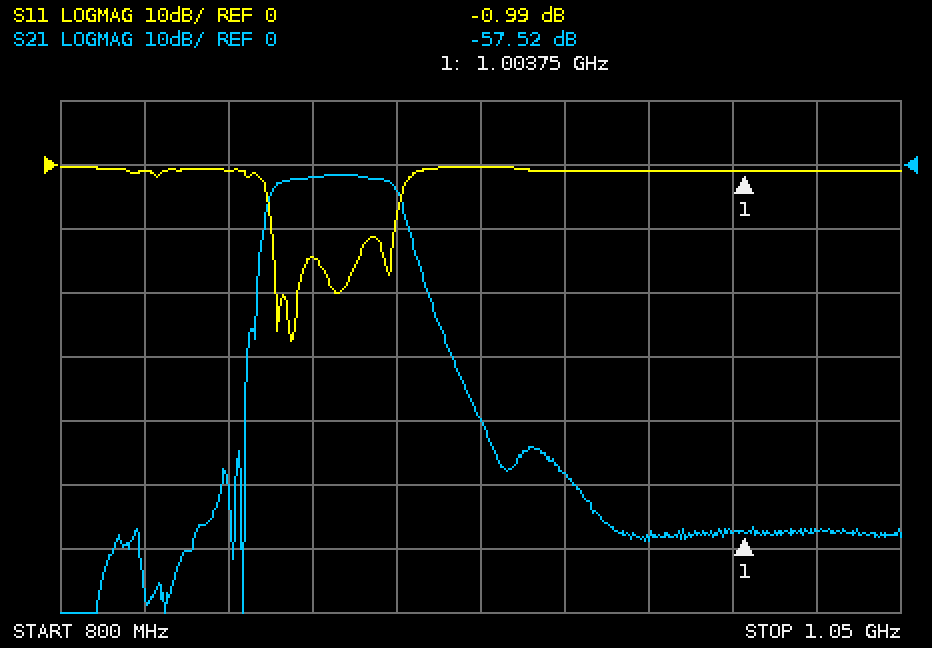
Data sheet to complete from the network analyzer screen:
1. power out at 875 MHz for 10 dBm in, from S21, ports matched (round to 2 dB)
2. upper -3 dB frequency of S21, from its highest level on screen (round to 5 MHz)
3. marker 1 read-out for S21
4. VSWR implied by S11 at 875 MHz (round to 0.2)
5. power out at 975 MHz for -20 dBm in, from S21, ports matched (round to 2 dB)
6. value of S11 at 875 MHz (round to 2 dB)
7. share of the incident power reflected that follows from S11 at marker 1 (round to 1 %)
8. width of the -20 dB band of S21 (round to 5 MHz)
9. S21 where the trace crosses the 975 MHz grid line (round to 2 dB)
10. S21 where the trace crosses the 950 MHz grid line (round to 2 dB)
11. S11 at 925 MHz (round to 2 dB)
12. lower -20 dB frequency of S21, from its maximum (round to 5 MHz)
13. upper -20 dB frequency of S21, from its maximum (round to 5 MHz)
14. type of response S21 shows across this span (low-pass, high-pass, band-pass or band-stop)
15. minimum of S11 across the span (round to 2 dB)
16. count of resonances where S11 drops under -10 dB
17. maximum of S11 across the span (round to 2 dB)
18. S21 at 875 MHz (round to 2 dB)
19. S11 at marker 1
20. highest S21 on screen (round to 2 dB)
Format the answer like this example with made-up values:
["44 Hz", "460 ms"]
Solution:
["8 dBm", "900 MHz", "-57.52 dB", "1.4", "-78 dBm", "-14 dB", "80 %", "50 MHz", "-58 dB", "-48 dB", "0 dB", "860 MHz", "910 MHz", "band-pass", "-28 dB", "4", "0 dB", "-2 dB", "-0.99 dB", "-2 dB"]
